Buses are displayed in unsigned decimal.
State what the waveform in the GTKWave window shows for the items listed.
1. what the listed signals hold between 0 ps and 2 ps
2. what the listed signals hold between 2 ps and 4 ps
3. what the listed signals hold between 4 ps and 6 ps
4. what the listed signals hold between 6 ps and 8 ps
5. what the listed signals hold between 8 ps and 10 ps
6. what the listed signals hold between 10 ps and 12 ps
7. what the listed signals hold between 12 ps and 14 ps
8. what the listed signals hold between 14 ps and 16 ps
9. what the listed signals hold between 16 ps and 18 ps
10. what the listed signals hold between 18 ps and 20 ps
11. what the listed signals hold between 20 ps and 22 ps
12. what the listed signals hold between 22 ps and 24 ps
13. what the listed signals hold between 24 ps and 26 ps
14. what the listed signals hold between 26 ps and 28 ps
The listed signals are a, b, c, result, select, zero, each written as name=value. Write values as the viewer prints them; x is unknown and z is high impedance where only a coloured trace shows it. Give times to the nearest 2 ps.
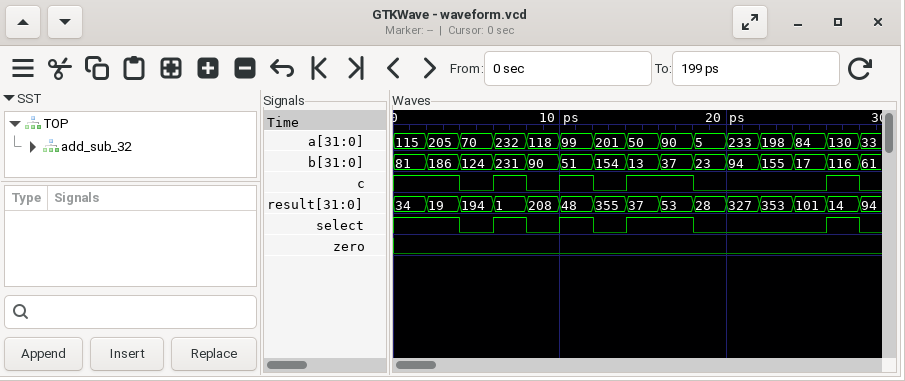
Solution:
a=115, b=81, c=1, result=34, select=1, zero=0
a=205, b=186, c=1, result=19, select=1, zero=0
a=70, b=124, c=0, result=194, select=0, zero=0
a=232, b=231, c=1, result=1, select=1, zero=0
a=118, b=90, c=0, result=208, select=0, zero=0
a=99, b=51, c=1, result=48, select=1, zero=0
a=201, b=154, c=0, result=355, select=0, zero=0
a=50, b=13, c=1, result=37, select=1, zero=0
a=90, b=37, c=1, result=53, select=1, zero=0
a=5, b=23, c=0, result=28, select=0, zero=0
a=233, b=94, c=0, result=327, select=0, zero=0
a=198, b=155, c=0, result=353, select=0, zero=0
a=84, b=17, c=0, result=101, select=0, zero=0
a=130, b=116, c=1, result=14, select=1, zero=0
